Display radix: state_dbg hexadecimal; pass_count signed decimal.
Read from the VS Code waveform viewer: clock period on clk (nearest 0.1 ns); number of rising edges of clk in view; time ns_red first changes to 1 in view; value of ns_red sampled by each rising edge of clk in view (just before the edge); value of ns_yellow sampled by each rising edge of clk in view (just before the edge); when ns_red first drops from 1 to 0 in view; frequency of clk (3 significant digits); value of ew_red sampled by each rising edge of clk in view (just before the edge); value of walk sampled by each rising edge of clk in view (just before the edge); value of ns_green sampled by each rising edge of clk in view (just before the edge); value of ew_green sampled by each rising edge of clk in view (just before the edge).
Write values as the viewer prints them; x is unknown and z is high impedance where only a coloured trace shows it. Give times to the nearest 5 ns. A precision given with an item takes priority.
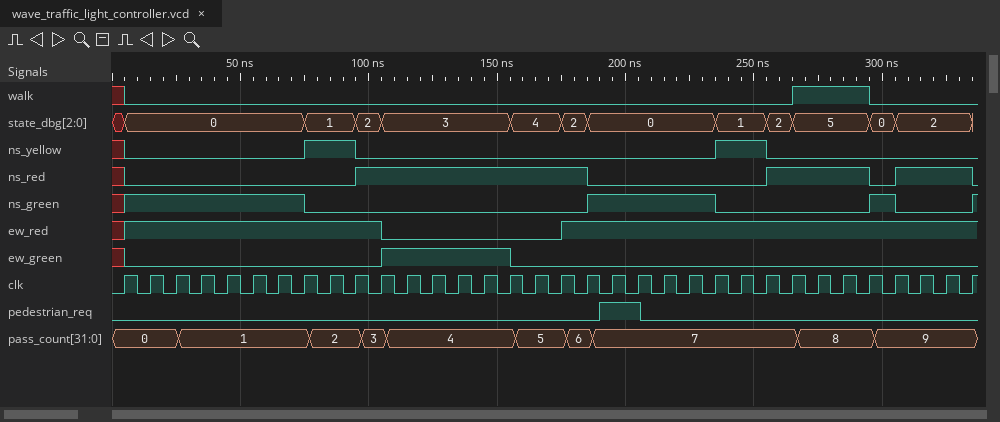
10 ns
34
95 ns
x 0 0 0 0 0 0 0 0 0 1 1 1 1 1 1 1 1 1 0 0 0 0 0 0 0 1 1 1 1 0 1 1 1
x 0 0 0 0 0 0 0 1 1 0 0 0 0 0 0 0 0 0 0 0 0 0 0 1 1 0 0 0 0 0 0 0 0
185 ns
100 MHz
x 1 1 1 1 1 1 1 1 1 1 0 0 0 0 0 0 0 1 1 1 1 1 1 1 1 1 1 1 1 1 1 1 1
x 0 0 0 0 0 0 0 0 0 0 0 0 0 0 0 0 0 0 0 0 0 0 0 0 0 0 1 1 1 0 0 0 0
x 1 1 1 1 1 1 1 0 0 0 0 0 0 0 0 0 0 0 1 1 1 1 1 0 0 0 0 0 0 1 0 0 0
x 0 0 0 0 0 0 0 0 0 0 1 1 1 1 1 0 0 0 0 0 0 0 0 0 0 0 0 0 0 0 0 0 0
